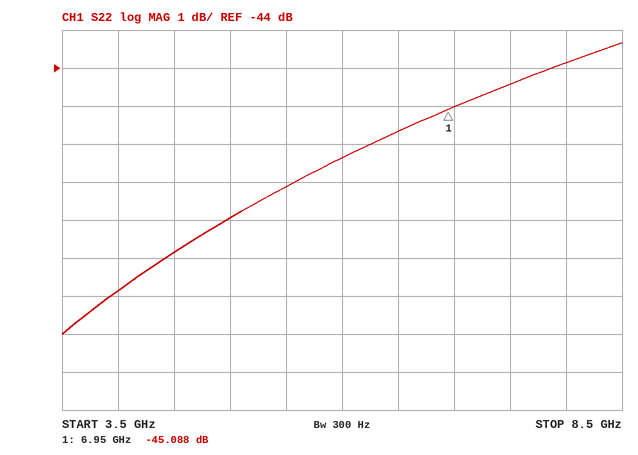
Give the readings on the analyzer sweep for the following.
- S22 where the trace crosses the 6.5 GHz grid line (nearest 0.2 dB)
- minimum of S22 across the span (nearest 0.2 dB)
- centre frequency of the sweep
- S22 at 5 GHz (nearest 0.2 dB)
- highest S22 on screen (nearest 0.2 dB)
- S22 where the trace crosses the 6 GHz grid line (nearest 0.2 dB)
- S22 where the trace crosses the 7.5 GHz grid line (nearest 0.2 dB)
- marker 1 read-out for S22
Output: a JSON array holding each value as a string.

["-45.6 dB", "-51.0 dB", "6 GHz", "-48.0 dB", "-43.4 dB", "-46.4 dB", "-44.4 dB", "-45.088 dB"]
